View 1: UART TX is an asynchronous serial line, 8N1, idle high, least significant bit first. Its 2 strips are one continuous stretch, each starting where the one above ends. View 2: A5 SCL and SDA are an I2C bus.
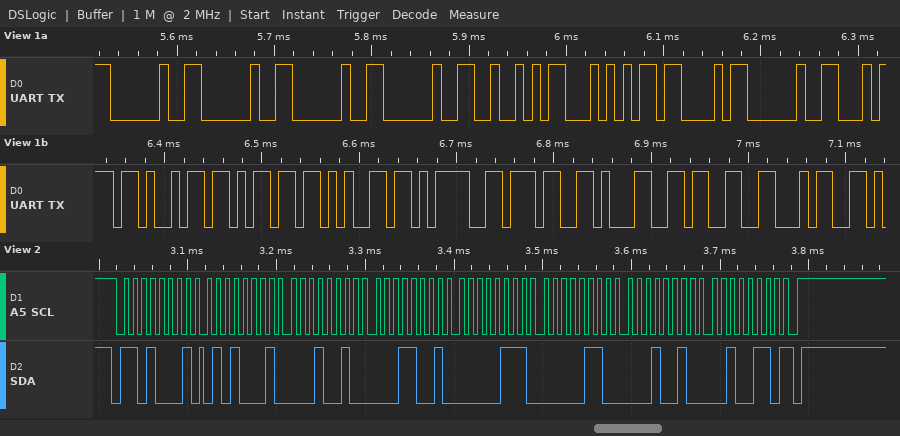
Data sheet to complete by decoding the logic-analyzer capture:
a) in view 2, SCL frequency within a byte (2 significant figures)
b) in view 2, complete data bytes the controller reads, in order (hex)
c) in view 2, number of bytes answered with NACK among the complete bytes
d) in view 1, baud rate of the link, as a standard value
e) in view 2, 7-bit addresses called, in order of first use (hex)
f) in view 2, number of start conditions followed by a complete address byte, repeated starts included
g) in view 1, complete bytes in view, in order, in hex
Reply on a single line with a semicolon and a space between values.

100 kHz; 51 12 19 07 06 12 26; 1; 115200 baud; 0x68; 1; 20 20 20 20 52 54 43 20 74 69 6D 65 3D 37 31 33 34
